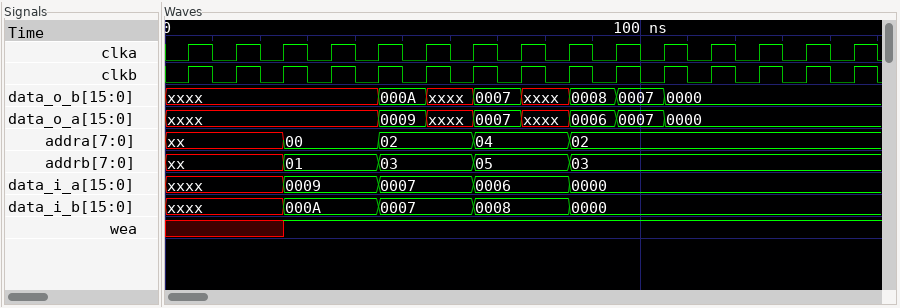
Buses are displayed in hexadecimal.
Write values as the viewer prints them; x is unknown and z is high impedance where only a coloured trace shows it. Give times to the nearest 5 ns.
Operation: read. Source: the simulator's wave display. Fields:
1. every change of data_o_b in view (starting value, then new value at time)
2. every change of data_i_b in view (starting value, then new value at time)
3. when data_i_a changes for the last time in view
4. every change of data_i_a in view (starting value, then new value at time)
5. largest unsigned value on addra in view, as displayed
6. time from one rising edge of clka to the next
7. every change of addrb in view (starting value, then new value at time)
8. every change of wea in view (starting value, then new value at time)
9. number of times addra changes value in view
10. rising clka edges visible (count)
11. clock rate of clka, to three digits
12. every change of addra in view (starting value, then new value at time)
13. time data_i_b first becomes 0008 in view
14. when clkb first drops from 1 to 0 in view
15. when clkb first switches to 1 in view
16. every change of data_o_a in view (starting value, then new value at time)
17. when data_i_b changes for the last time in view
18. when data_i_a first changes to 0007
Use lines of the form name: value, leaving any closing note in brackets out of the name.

every change of data_o_b in view: xxxx, 000A at 45 ns, xxxx at 55 ns, 0007 at 65 ns, xxxx at 75 ns, 0008 at 85 ns, 0007 at 95 ns, 0000 at 105 ns
every change of data_i_b in view: xxxx, 000A at 25 ns, 0007 at 45 ns, 0008 at 65 ns, 0000 at 85 ns
when data_i_a changes for the last time in view: 85 ns
every change of data_i_a in view: xxxx, 0009 at 25 ns, 0007 at 45 ns, 0006 at 65 ns, 0000 at 85 ns
largest unsigned value on addra in view, as displayed: 04
time from one rising edge of clka to the next: 10 ns
every change of addrb in view: xx, 01 at 25 ns, 03 at 45 ns, 05 at 65 ns, 03 at 85 ns
every change of wea in view: x, 1 at 25 ns
number of times addra changes value in view: 4
rising clka edges visible: 15
clock rate of clka, to three digits: 100 MHz
every change of addra in view: xx, 00 at 25 ns, 02 at 45 ns, 04 at 65 ns, 02 at 85 ns
time data_i_b first becomes 0008 in view: 65 ns
when clkb first drops from 1 to 0 in view: 10 ns
when clkb first switches to 1 in view: 5 ns
every change of data_o_a in view: xxxx, 0009 at 45 ns, xxxx at 55 ns, 0007 at 65 ns, xxxx at 75 ns, 0006 at 85 ns, 0007 at 95 ns, 0000 at 105 ns
when data_i_b changes for the last time in view: 85 ns
when data_i_a first changes to 0007: 45 ns
